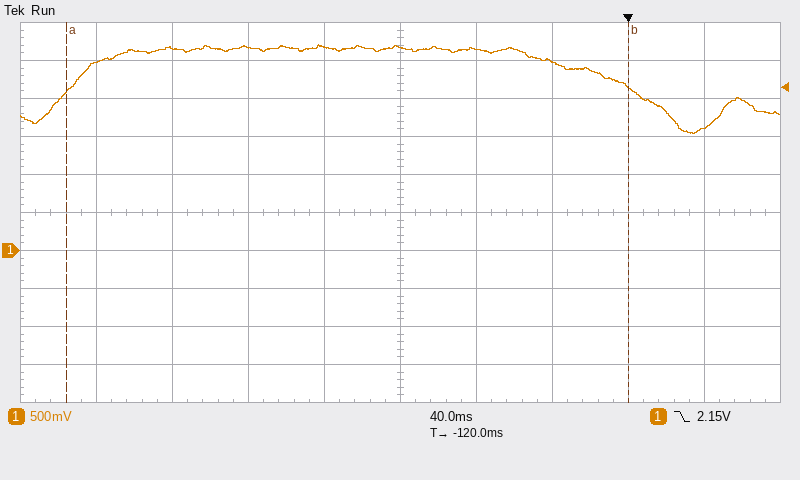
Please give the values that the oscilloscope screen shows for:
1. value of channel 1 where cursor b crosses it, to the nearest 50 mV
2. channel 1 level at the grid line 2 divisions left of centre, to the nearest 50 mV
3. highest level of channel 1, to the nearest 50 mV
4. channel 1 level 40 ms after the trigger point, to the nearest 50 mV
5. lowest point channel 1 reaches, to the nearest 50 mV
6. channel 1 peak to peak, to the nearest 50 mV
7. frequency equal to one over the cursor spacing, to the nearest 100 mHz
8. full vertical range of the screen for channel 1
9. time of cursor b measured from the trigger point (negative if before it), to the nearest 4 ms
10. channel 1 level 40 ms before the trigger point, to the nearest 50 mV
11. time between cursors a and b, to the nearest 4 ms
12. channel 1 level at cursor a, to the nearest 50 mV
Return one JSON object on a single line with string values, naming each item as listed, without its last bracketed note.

{"value of channel 1 where cursor b crosses it, to the nearest 50 mV": "2.15 V", "channel 1 level at the grid line 2 divisions left of centre, to the nearest 50 mV": "2.70 V", "highest level of channel 1, to the nearest 50 mV": "2.70 V", "channel 1 level 40 ms after the trigger point, to the nearest 50 mV": "1.60 V", "lowest point channel 1 reaches, to the nearest 50 mV": "1.55 V", "channel 1 peak to peak, to the nearest 50 mV": "1.15 V", "frequency equal to one over the cursor spacing, to the nearest 100 mHz": "3.4 Hz", "full vertical range of the screen for channel 1": "5 V", "time of cursor b measured from the trigger point (negative if before it), to the nearest 4 ms": "0 ms", "channel 1 level 40 ms before the trigger point, to the nearest 50 mV": "2.50 V", "time between cursors a and b, to the nearest 4 ms": "296 ms", "channel 1 level at cursor a, to the nearest 50 mV": "2.10 V"}
